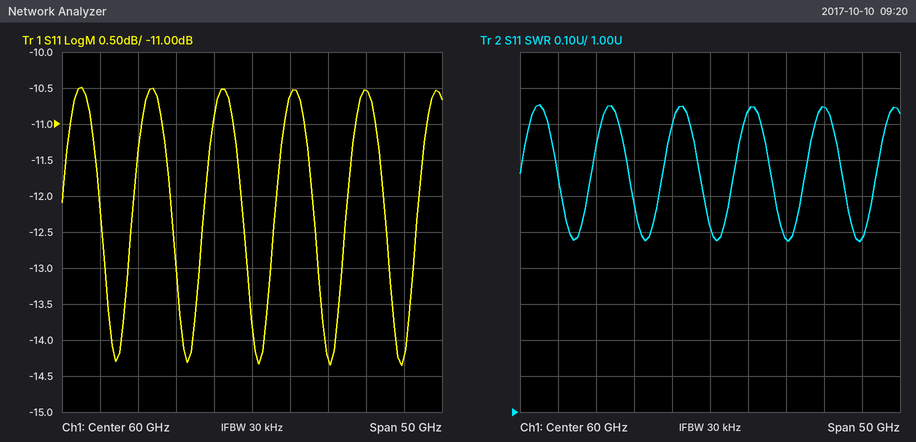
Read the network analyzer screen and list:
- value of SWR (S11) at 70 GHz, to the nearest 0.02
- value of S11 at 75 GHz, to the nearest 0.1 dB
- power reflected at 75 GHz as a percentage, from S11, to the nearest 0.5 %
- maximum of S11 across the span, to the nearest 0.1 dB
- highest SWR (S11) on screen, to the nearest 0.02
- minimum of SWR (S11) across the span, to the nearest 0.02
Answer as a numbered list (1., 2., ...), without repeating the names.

1. 1.48
2. -10.5 dB
3. 9.0 %
4. -10.5 dB
5. 1.86
6. 1.48
